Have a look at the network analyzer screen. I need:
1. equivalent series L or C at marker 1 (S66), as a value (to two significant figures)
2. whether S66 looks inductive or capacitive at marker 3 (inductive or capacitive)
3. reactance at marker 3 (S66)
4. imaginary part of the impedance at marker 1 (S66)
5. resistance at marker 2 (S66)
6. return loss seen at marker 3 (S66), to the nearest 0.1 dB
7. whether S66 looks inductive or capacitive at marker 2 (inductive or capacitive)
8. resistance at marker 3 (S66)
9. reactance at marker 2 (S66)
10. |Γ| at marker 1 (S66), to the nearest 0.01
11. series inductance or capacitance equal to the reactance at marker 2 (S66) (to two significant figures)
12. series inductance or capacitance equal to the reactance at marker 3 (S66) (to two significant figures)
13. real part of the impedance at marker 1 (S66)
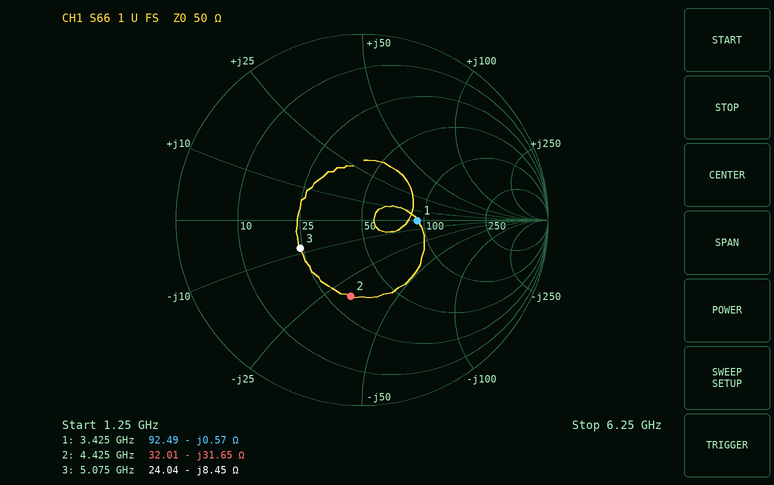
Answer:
82 pF
capacitive
-8.45 Ω
-0.57 Ω
32.01 Ω
8.7 dB
capacitive
24.04 Ω
-31.65 Ω
0.30
1.1 pF
3.7 pF
92.49 Ω
